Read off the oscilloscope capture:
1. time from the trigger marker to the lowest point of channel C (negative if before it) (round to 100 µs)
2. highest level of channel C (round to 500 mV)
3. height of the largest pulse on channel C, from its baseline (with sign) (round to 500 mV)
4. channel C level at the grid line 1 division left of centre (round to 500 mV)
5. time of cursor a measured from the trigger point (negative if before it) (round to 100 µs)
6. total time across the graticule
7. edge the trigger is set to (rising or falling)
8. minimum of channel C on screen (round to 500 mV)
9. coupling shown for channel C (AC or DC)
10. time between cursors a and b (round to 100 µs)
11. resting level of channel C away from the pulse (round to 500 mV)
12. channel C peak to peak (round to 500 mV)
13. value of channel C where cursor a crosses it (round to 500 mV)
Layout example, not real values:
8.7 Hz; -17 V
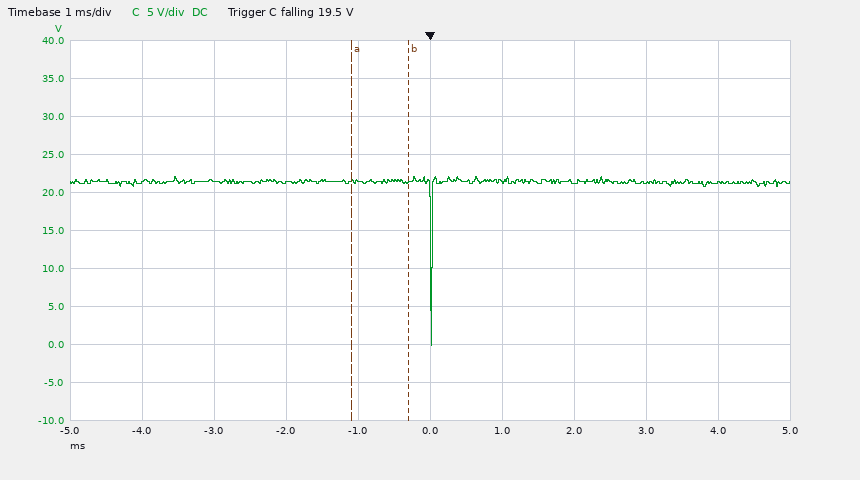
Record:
0.0 ms; 22.0 V; -21.5 V; 21.5 V; -1.1 ms; 10 ms; falling; 0.0 V; DC; 800 µs; 21.5 V; 22.0 V; 21.5 V
